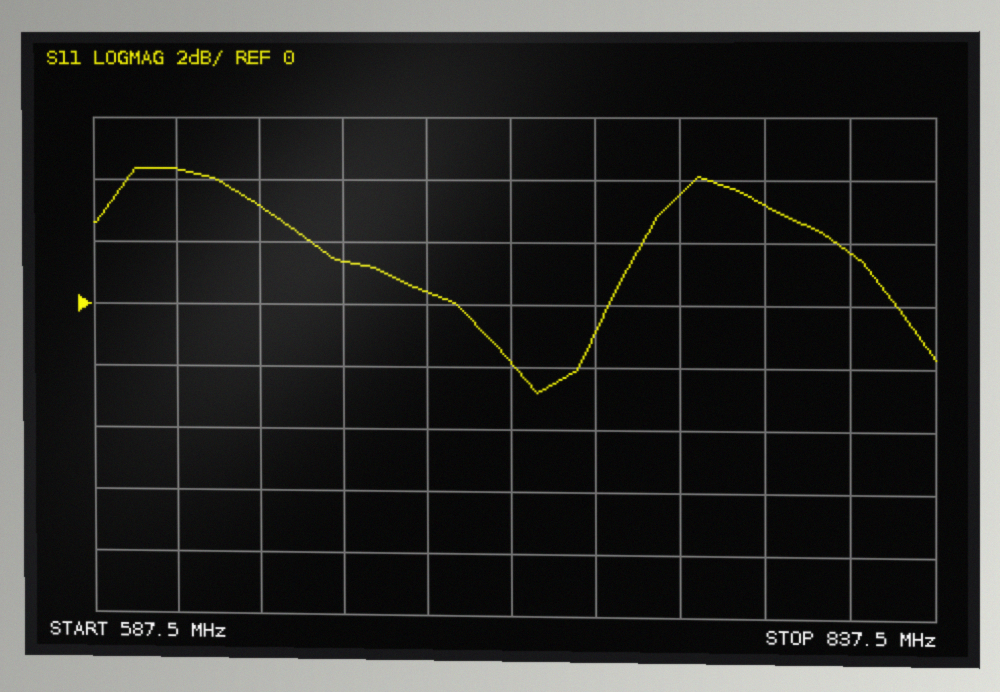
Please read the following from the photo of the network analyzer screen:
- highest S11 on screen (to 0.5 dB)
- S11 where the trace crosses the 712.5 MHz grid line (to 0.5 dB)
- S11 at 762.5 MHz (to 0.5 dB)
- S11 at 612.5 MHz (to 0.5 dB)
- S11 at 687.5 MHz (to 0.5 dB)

4.5 dB
-2.0 dB
3.5 dB
4.5 dB
0.5 dB
